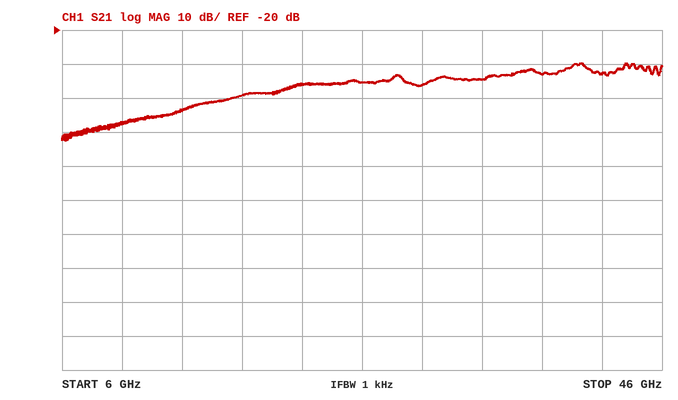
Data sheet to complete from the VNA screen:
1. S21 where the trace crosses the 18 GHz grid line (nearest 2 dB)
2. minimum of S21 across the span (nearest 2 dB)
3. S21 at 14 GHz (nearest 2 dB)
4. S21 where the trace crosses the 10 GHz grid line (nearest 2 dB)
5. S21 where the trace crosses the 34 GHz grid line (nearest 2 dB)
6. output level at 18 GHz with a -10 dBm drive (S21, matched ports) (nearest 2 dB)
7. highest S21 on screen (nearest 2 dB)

-40 dB
-52 dB
-44 dB
-48 dB
-34 dB
-50 dBm
-30 dB
